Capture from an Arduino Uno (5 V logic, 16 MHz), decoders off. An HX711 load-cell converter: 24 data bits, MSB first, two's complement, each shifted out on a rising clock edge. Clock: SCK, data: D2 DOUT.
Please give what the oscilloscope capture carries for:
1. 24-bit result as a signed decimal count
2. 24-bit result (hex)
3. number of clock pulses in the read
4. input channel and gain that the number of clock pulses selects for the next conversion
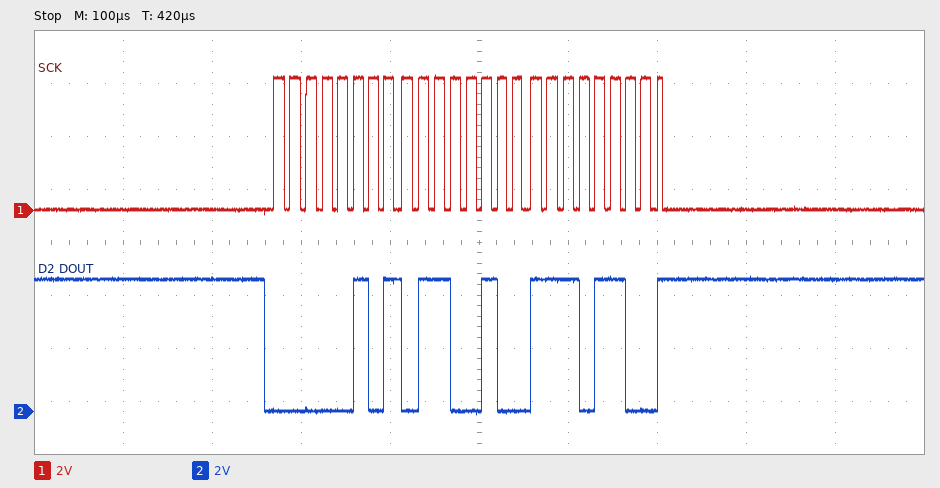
353516
0x0564EC
25
channel A, gain 128
